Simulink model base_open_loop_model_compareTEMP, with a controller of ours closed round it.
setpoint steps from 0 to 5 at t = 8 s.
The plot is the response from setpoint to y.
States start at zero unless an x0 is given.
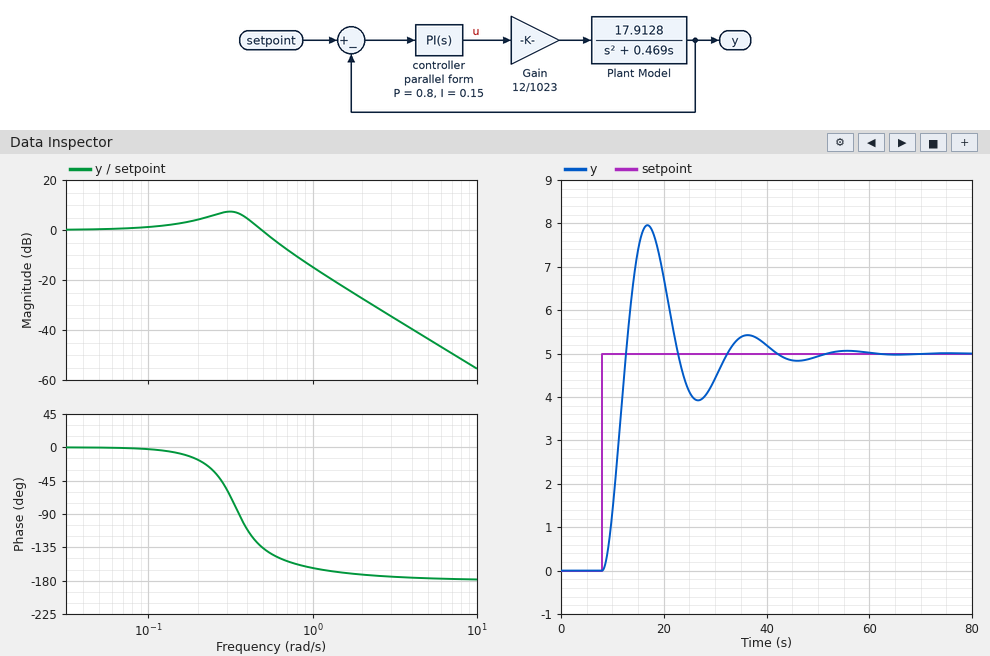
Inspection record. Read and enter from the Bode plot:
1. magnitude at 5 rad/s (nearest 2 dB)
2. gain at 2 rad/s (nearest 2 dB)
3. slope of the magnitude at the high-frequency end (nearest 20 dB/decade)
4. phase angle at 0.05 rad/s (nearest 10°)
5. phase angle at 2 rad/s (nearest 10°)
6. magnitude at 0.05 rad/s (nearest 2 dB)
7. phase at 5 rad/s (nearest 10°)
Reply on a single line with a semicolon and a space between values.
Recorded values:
-44 dB; -28 dB; -40 dB/decade; 0°; -170°; 0 dB; -180°
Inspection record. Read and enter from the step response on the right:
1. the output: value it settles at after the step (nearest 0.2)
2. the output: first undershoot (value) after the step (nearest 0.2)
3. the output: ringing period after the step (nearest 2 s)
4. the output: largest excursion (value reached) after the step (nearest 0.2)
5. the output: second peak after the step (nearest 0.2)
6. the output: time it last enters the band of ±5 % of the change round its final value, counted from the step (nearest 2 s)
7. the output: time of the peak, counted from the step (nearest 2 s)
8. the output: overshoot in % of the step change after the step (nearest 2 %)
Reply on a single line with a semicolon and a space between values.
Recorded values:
5.0; 4.0; 20 s; 8.0; 5.4; 32 s; 8 s; 60 %
